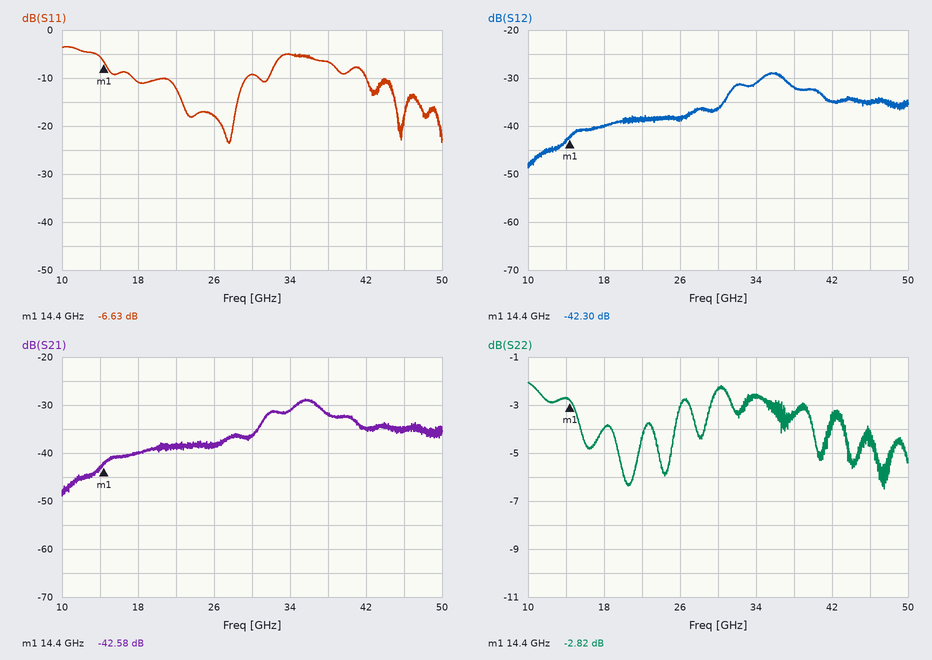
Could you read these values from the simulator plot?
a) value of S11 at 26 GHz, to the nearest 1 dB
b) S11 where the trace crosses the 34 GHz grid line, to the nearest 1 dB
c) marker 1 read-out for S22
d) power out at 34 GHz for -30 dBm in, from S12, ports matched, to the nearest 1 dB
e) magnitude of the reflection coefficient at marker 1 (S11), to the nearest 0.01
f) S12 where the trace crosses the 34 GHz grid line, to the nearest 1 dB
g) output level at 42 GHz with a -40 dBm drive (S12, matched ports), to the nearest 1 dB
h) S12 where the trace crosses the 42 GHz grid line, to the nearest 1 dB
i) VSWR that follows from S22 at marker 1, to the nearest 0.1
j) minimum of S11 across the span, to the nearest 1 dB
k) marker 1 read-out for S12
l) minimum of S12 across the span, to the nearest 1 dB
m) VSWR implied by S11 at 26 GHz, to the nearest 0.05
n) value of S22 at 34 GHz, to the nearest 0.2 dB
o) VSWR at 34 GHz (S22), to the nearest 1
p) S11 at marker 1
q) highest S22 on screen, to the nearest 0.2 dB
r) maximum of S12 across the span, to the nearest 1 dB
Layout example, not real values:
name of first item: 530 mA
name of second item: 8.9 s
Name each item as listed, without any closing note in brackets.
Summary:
value of S11 at 26 GHz, to the nearest 1 dB: -18 dB
S11 where the trace crosses the 34 GHz grid line, to the nearest 1 dB: -5 dB
marker 1 read-out for S22: -2.82 dB
power out at 34 GHz for -30 dBm in, from S12, ports matched, to the nearest 1 dB: -61 dBm
magnitude of the reflection coefficient at marker 1 (S11), to the nearest 0.01: 0.47
S12 where the trace crosses the 34 GHz grid line, to the nearest 1 dB: -31 dB
output level at 42 GHz with a -40 dBm drive (S12, matched ports), to the nearest 1 dB: -75 dBm
S12 where the trace crosses the 42 GHz grid line, to the nearest 1 dB: -35 dB
VSWR that follows from S22 at marker 1, to the nearest 0.1: 6.2
minimum of S11 across the span, to the nearest 1 dB: -24 dB
marker 1 read-out for S12: -42.30 dB
minimum of S12 across the span, to the nearest 1 dB: -49 dB
VSWR implied by S11 at 26 GHz, to the nearest 0.05: 1.30
value of S22 at 34 GHz, to the nearest 0.2 dB: -2.6 dB
VSWR at 34 GHz (S22), to the nearest 1: 7
S11 at marker 1: -6.63 dB
highest S22 on screen, to the nearest 0.2 dB: -2.0 dB
maximum of S12 across the span, to the nearest 1 dB: -29 dB
